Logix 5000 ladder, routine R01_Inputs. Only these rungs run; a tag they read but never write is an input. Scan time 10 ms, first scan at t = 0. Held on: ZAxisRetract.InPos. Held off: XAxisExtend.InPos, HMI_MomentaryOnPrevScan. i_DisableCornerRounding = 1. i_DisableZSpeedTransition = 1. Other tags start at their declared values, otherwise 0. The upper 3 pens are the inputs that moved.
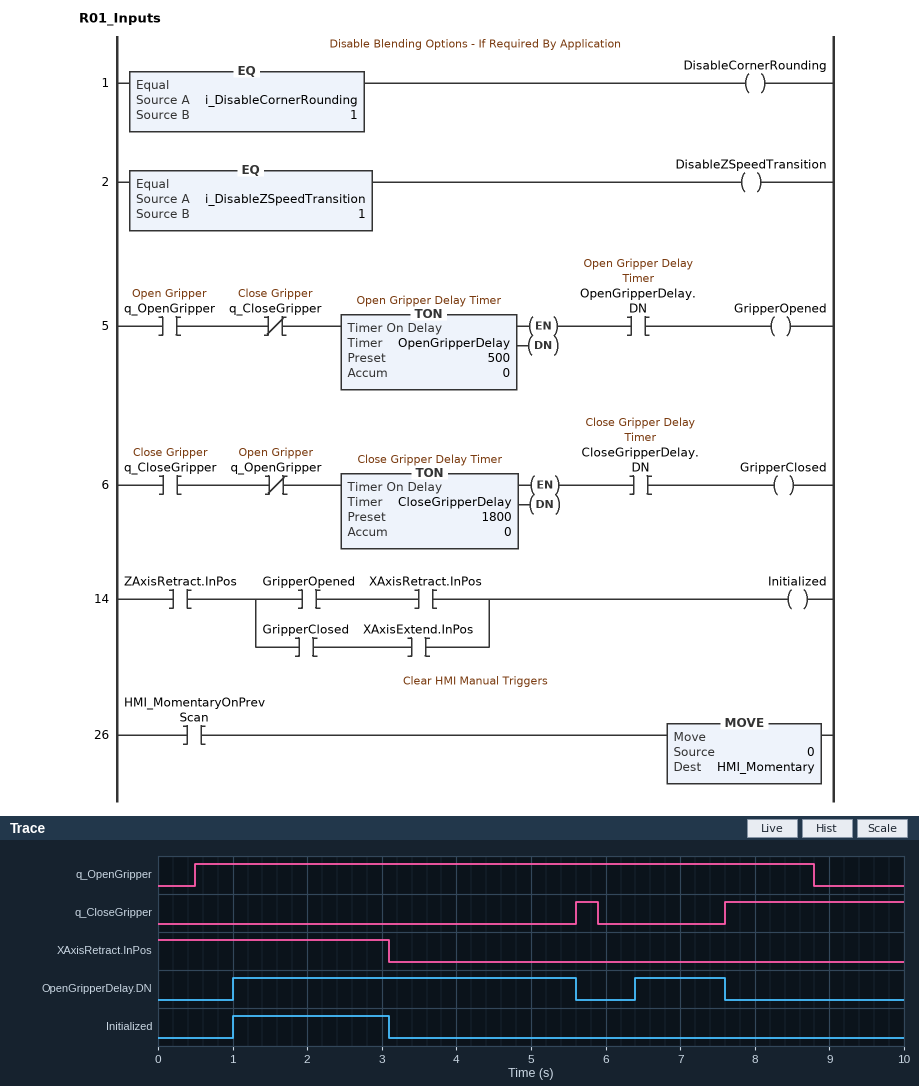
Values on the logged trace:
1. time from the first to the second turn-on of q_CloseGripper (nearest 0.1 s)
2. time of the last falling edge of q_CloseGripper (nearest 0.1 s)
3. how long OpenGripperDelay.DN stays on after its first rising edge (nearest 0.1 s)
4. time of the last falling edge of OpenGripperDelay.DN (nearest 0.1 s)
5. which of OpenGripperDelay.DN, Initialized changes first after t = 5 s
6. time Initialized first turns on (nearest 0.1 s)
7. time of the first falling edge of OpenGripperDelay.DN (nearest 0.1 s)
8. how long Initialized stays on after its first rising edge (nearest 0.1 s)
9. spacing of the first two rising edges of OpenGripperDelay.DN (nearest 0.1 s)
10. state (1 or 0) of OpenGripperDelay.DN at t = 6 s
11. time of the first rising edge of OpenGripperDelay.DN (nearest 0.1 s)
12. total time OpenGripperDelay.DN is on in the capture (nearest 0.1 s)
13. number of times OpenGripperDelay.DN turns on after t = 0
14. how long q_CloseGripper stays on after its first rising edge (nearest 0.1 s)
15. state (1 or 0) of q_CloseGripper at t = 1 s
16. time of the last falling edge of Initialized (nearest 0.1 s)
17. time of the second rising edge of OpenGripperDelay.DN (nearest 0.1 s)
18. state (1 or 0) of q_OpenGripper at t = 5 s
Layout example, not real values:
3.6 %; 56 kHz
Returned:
2.0 s; 5.9 s; 4.6 s; 7.6 s; OpenGripperDelay.DN; 1.0 s; 5.6 s; 2.1 s; 5.4 s; 0; 1.0 s; 5.8 s; 2; 0.3 s; 0; 3.1 s; 6.4 s; 1
